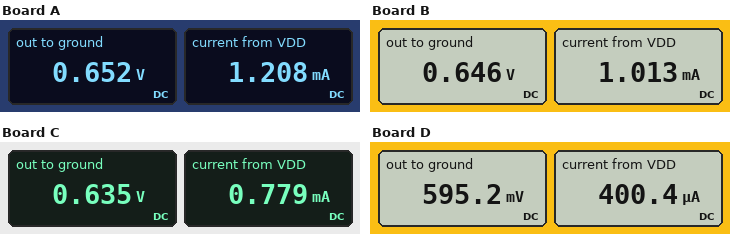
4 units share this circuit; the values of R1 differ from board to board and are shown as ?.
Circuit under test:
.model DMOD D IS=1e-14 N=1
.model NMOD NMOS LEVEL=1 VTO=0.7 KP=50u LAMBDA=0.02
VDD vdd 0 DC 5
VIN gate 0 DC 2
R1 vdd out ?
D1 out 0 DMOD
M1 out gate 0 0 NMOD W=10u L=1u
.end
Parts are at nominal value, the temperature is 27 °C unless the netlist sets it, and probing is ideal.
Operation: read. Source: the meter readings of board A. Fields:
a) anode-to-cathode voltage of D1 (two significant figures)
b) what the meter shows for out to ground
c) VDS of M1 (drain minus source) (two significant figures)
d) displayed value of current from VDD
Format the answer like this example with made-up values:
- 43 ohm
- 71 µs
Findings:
- 650 mV
- 0.652 V
- 650 mV
- 1.208 mA
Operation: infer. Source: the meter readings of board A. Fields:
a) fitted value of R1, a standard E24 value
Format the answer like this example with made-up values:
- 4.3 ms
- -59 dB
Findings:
- 3.6 kΩ
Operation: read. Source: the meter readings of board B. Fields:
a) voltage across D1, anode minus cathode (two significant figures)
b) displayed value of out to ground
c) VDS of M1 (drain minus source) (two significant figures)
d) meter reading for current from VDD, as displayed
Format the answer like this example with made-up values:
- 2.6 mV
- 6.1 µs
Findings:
- 650 mV
- 0.646 V
- 650 mV
- 1.013 mA
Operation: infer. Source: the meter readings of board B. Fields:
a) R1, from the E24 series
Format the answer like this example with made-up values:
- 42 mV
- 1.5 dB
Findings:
- 4.3 kΩ
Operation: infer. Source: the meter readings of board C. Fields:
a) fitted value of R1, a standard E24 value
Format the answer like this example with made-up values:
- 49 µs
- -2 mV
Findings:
- 5.6 kΩ
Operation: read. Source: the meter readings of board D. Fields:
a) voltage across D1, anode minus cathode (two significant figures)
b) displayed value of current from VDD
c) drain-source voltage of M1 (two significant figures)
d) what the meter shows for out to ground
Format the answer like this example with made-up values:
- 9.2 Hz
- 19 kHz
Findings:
- 600 mV
- 400.4 µA
- 600 mV
- 595.2 mV
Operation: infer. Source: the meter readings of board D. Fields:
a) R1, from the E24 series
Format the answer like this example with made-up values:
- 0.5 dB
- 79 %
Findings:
- 11 kΩ
